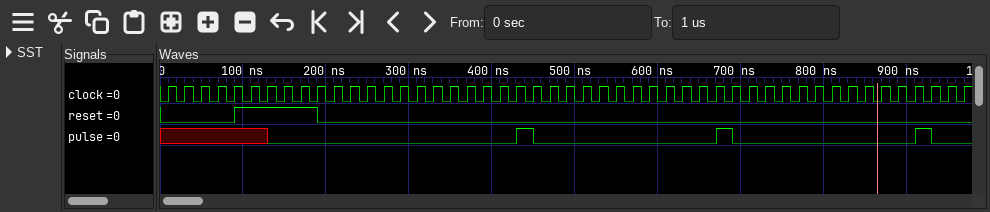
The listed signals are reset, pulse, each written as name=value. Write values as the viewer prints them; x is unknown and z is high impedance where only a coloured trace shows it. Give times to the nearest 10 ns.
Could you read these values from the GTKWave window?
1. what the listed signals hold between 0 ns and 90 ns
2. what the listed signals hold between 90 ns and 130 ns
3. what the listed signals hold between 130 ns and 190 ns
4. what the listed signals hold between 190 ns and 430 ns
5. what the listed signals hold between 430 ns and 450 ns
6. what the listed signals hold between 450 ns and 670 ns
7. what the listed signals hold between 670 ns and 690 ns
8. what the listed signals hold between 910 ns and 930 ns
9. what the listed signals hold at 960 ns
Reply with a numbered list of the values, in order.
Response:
1. reset=0, pulse=x
2. reset=1, pulse=x
3. reset=1, pulse=0
4. reset=0, pulse=0
5. reset=0, pulse=1
6. reset=0, pulse=0
7. reset=0, pulse=1
8. reset=0, pulse=1
9. reset=0, pulse=0
